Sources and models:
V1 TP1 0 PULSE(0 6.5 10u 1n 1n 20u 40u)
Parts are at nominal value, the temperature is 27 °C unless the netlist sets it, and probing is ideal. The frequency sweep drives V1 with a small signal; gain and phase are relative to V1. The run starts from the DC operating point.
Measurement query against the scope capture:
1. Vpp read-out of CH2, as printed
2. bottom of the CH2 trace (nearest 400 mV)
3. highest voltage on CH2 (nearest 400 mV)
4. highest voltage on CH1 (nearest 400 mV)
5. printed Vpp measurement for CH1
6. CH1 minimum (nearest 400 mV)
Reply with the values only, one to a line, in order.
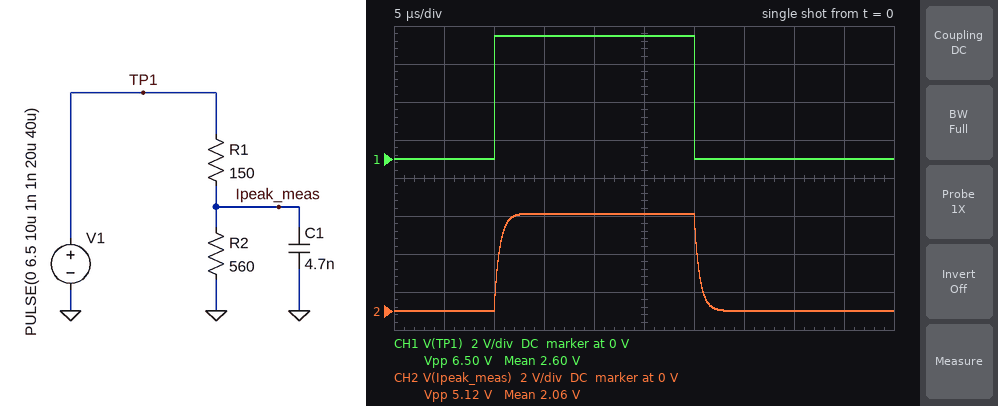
5.12 V
0 V
5.2 V
6.4 V
6.50 V
0 V
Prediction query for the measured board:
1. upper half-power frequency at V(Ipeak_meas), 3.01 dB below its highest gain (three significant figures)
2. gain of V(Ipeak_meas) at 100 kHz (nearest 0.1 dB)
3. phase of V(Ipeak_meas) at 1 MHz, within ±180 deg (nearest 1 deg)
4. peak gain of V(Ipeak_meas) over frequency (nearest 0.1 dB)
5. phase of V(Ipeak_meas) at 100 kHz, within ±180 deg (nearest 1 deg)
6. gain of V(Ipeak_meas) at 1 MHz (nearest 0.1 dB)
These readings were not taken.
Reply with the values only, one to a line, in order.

286 kHz
-2.6 dB
-74 deg
-2.1 dB
-19 deg
-13.3 dB
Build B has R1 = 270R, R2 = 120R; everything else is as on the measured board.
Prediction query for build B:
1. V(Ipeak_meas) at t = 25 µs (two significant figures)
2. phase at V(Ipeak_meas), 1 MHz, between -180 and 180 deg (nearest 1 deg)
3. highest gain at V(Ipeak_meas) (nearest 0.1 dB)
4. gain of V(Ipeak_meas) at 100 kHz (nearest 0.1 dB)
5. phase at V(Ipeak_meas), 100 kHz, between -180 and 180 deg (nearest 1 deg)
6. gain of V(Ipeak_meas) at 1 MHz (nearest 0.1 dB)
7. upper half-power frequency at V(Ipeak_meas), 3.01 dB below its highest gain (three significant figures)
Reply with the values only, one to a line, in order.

2.0 V
-68 deg
-10.2 dB
-10.5 dB
-14 deg
-18.7 dB
408 kHz
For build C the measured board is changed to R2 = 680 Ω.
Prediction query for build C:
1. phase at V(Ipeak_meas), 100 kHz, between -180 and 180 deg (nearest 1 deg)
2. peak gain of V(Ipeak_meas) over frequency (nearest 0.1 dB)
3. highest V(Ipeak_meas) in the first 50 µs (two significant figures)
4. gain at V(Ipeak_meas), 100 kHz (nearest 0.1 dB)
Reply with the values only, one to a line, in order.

-20 deg
-1.7 dB
5.3 V
-2.3 dB
